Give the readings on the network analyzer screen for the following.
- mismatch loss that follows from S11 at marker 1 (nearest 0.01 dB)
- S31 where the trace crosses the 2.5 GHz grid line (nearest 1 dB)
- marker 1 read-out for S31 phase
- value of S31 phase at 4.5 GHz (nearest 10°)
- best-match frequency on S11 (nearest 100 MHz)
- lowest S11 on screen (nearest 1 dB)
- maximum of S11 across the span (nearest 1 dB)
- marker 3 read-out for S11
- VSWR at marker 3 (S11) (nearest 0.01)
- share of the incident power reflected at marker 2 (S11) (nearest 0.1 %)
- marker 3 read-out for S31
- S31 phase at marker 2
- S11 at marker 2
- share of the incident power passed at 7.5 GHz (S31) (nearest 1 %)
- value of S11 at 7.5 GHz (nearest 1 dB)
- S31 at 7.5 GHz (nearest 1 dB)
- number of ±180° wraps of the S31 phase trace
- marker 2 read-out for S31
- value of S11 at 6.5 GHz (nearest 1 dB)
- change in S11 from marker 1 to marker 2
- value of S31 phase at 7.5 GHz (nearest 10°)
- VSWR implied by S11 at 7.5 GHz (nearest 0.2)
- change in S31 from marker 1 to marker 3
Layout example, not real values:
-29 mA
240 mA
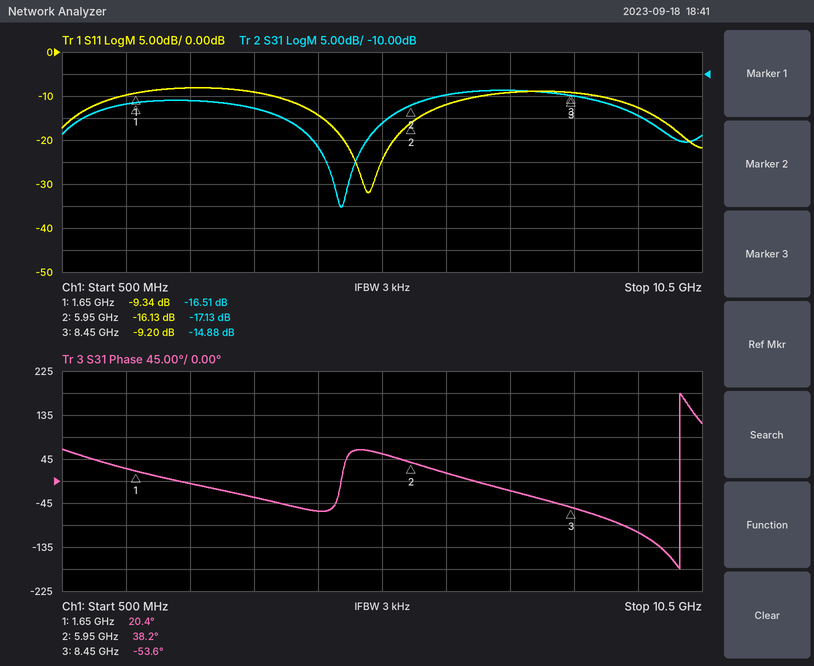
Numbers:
0.54 dB
-16 dB
20.4°
-60°
5.3 GHz
-32 dB
-8 dB
-9.20 dB
2.06
2.4 %
-14.88 dB
38.2°
-16.13 dB
4 %
-9 dB
-14 dB
1
-17.13 dB
-12 dB
-6.79 dB
-20°
2.0
1.63 dB
